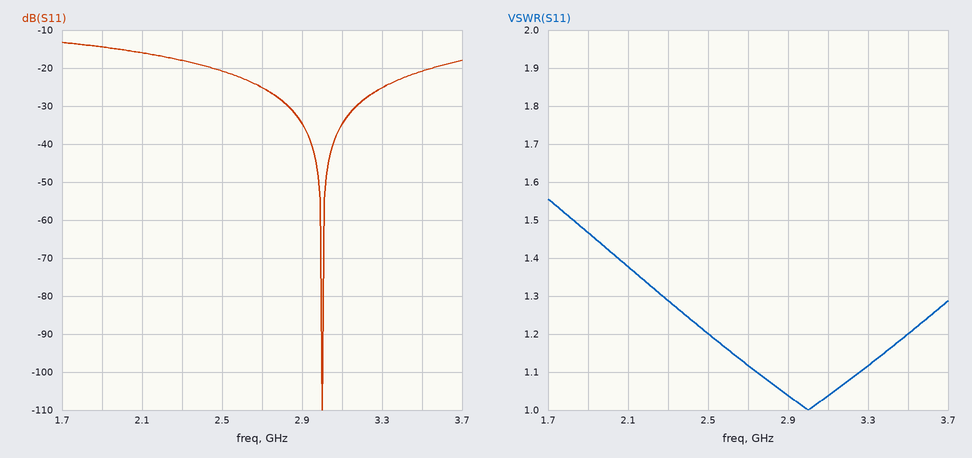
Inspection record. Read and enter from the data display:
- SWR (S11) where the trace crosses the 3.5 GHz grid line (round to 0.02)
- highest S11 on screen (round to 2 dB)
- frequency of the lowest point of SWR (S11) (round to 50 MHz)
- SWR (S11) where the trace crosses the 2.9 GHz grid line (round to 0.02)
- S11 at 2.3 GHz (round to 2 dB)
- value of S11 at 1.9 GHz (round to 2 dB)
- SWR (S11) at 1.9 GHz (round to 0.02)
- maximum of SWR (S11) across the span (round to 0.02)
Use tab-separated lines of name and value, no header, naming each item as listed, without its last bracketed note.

SWR (S11) where the trace crosses the 3.5 GHz grid line	1.20
highest S11 on screen	-14 dB
frequency of the lowest point of SWR (S11)	3.00 GHz
SWR (S11) where the trace crosses the 2.9 GHz grid line	1.04
S11 at 2.3 GHz	-18 dB
value of S11 at 1.9 GHz	-14 dB
SWR (S11) at 1.9 GHz	1.46
maximum of SWR (S11) across the span	1.56
